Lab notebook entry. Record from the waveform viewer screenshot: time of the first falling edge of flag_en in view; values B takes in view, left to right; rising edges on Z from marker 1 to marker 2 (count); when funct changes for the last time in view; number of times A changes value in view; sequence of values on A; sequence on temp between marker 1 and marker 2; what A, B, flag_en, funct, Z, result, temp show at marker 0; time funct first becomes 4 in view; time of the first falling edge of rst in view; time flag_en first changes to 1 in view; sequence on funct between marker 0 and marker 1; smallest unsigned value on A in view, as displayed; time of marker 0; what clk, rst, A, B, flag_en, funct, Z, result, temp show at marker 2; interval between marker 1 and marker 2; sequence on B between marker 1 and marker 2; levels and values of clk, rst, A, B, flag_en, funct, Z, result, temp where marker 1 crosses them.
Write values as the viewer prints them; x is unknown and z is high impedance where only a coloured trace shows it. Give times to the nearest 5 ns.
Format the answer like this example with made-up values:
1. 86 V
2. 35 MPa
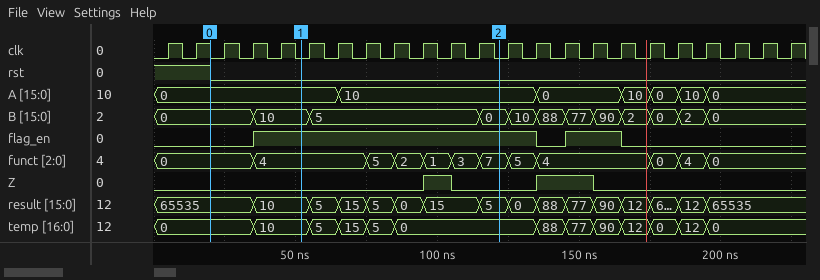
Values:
1. 135 ns
2. 0, 10, 5, 0, 10, 88, 77, 90, 2, 0, 2, 0
3. 1
4. 195 ns
5. 6
6. 0, 10, 0, 10, 0, 10, 0
7. 10, 5, 15, 5, 0
8. A=0, B=0, flag_en=0, funct=0, Z=0, result=65535, temp=0
9. 35 ns
10. 20 ns
11. 35 ns
12. 0, 4
13. 0
14. 20 ns
15. clk=0, rst=0, A=10, B=0, flag_en=1, funct=7, Z=0, result=5, temp=0
16. 70 ns
17. 10, 5, 0
18. clk=0, rst=0, A=0, B=10, flag_en=1, funct=4, Z=0, result=10, temp=10
